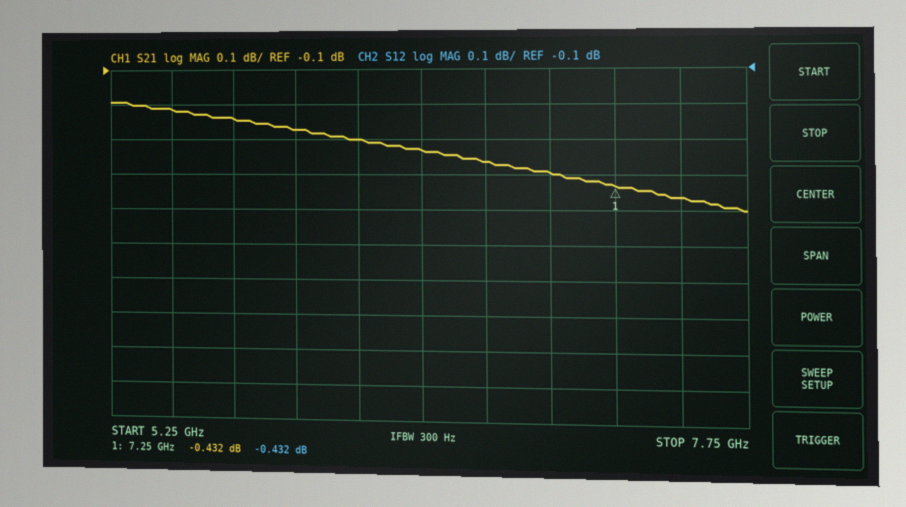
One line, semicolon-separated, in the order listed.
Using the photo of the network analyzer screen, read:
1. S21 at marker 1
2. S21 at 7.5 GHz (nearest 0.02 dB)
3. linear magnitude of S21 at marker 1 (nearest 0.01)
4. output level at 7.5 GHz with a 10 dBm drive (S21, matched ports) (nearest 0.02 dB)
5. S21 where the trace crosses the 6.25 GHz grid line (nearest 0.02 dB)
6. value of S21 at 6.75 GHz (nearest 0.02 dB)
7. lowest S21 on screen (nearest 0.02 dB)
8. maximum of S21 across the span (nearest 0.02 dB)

-0.432 dB; -0.46 dB; 0.95; 9.54 dBm; -0.30 dB; -0.36 dB; -0.50 dB; -0.20 dB
